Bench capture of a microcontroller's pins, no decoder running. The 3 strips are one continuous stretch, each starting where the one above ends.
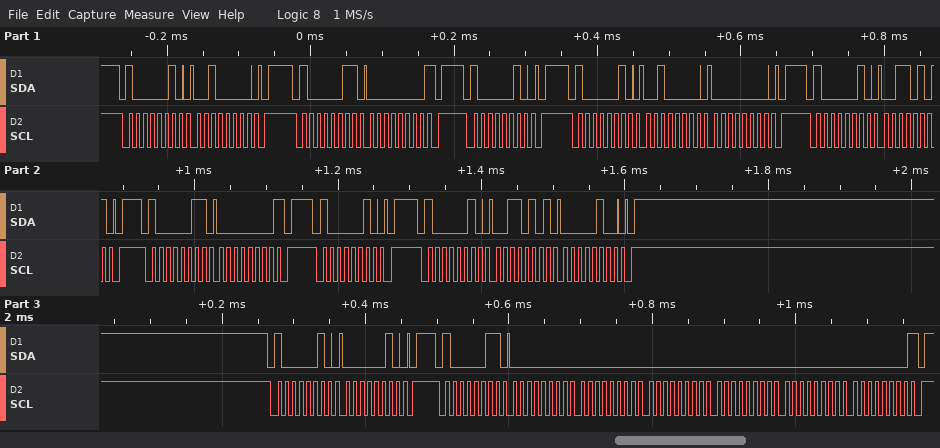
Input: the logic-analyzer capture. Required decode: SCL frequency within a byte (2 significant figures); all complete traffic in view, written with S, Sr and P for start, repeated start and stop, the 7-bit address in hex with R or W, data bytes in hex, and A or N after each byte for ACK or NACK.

100 kHz
S 41W A 20 A P S 41R A 00 N P S 41W A P S 41W A 20 A 00 A P S 41W A 35 A P S 41R A 00 N P S 41W A P S 41W A 35 A 04 A P S 41W A 02 A P S 41R A 00 A 00 A 00 A 00 A 00 A 00 N P
